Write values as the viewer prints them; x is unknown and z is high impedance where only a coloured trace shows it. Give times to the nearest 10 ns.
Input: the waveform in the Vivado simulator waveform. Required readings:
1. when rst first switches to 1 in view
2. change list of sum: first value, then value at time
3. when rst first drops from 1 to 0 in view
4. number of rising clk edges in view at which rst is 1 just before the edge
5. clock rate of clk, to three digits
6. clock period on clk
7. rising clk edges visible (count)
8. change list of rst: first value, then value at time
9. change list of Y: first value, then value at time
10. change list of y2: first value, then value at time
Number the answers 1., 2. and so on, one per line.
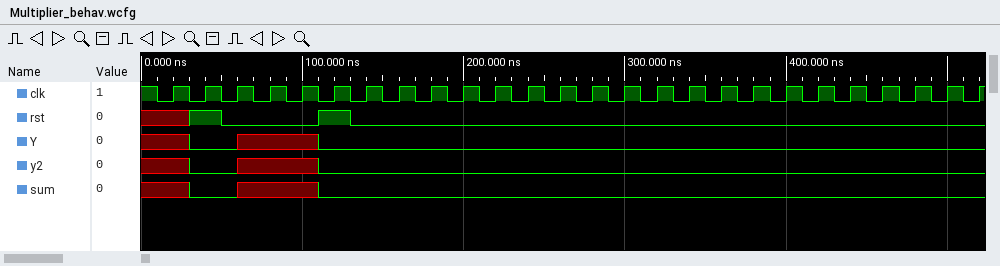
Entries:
1. 30 ns
2. x, 0 at 30 ns, x at 60 ns, 0 at 110 ns
3. 50 ns
4. 2
5. 50.0 MHz
6. 20 ns
7. 26
8. x, 1 at 30 ns, 0 at 50 ns, 1 at 110 ns, 0 at 130 ns
9. x, 0 at 30 ns, x at 60 ns, 0 at 110 ns
10. x, 0 at 30 ns, x at 60 ns, 0 at 110 ns
